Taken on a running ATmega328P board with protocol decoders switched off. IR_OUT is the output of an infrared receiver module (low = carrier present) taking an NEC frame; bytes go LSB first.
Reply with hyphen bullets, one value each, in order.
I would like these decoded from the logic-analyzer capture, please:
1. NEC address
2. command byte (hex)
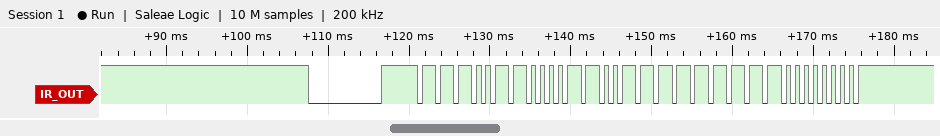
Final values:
- 0x67
- 0xFF
